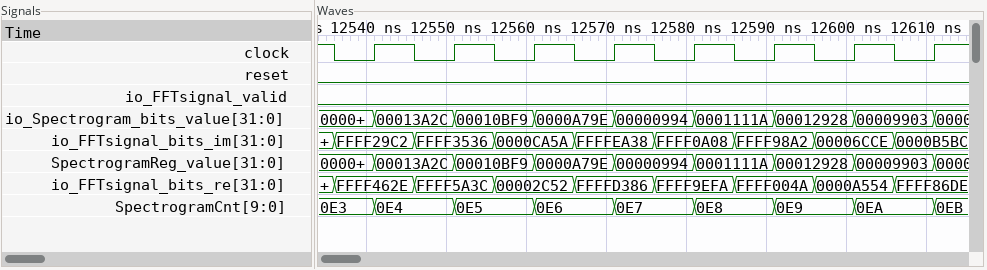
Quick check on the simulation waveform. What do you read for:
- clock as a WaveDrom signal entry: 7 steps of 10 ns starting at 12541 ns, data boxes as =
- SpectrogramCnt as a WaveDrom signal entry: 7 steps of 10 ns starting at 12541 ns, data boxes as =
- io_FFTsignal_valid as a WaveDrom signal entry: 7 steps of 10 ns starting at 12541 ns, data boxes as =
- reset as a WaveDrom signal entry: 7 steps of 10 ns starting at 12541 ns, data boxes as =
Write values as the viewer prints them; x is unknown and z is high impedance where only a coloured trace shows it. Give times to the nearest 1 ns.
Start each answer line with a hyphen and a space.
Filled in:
- {name: 'clock', wave: 'p......'}
- {name: 'SpectrogramCnt', wave: '=======', data: '0E4 0E5 0E6 0E7 0E8 0E9 0EA'}
- {name: 'io_FFTsignal_valid', wave: '0......'}
- {name: 'reset', wave: '0......'}
